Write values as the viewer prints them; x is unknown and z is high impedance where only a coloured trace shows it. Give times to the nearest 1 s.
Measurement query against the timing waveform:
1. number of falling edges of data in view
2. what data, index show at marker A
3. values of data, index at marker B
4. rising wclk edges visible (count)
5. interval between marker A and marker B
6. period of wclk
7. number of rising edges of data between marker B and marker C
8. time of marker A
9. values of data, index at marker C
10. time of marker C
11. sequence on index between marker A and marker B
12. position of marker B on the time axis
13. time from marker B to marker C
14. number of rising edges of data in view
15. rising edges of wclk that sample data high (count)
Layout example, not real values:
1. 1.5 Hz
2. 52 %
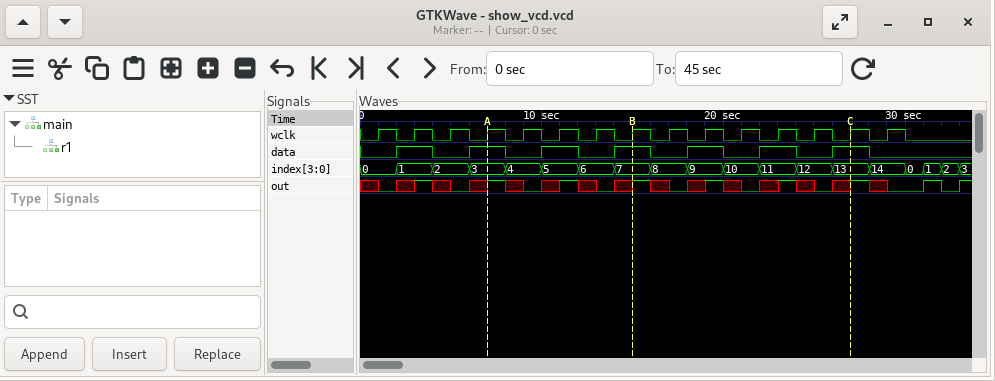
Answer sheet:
1. 7
2. data=1, index=3
3. data=1, index=7
4. 15
5. 8 s
6. 2 s
7. 3
8. 7 s
9. data=1, index=13
10. 27 s
11. 3, 4, 5, 6, 7
12. 15 s
13. 12 s
14. 7
15. 7
